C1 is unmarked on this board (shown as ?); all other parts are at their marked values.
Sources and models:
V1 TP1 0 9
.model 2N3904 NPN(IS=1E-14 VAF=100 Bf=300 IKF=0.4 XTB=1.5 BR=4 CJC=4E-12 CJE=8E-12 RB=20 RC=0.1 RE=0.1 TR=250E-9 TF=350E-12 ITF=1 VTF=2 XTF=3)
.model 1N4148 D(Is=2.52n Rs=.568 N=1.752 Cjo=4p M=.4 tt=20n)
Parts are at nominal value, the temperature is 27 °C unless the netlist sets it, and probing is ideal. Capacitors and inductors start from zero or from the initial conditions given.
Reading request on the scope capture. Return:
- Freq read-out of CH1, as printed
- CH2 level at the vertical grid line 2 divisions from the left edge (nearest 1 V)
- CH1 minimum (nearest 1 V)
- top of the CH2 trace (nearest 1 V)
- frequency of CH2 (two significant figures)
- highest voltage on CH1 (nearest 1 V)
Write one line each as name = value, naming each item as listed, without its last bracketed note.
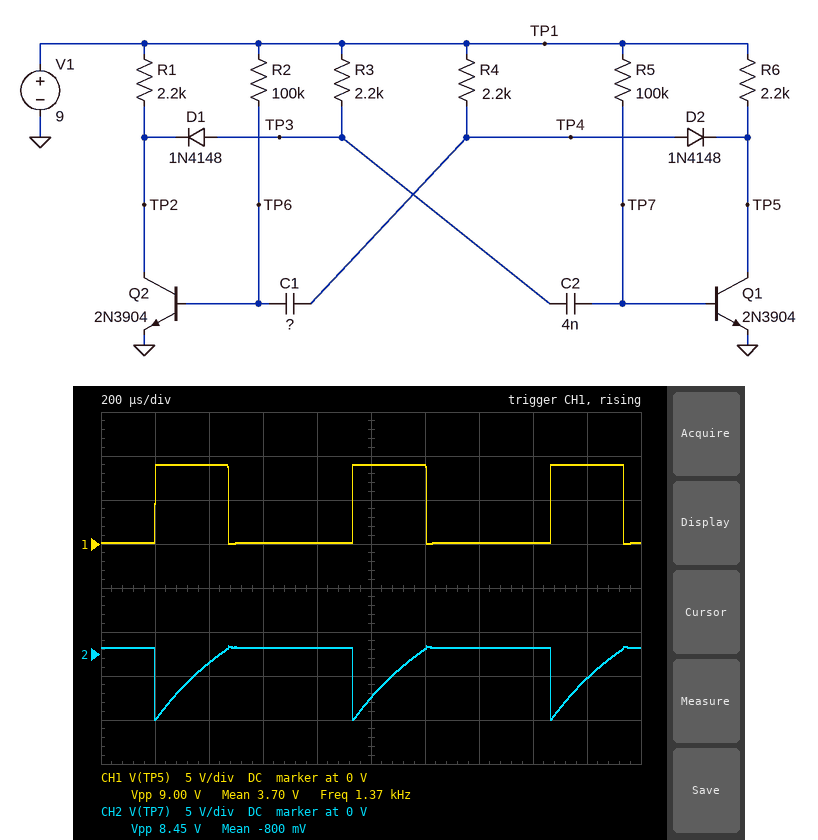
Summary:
Freq read-out of CH1, as printed = 1.37 kHz
CH2 level at the vertical grid line 2 divisions from the left edge = -1 V
CH1 minimum = 0 V
top of the CH2 trace = 1 V
frequency of CH2 = 1.4 kHz
highest voltage on CH1 = 9 V
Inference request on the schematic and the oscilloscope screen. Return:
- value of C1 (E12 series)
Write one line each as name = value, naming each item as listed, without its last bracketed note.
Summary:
value of C1 = 6.8 nF
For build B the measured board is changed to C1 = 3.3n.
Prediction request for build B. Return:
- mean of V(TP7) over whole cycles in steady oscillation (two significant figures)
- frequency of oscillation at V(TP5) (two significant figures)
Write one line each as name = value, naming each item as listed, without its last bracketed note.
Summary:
mean of V(TP7) over whole cycles in steady oscillation = -1.3 V
frequency of oscillation at V(TP5) = 2.0 kHz
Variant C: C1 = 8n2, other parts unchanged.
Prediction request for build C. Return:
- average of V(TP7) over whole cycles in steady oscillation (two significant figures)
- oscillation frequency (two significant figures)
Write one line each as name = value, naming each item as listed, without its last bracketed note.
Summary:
average of V(TP7) over whole cycles in steady oscillation = -500 mV
oscillation frequency = 1.2 kHz
